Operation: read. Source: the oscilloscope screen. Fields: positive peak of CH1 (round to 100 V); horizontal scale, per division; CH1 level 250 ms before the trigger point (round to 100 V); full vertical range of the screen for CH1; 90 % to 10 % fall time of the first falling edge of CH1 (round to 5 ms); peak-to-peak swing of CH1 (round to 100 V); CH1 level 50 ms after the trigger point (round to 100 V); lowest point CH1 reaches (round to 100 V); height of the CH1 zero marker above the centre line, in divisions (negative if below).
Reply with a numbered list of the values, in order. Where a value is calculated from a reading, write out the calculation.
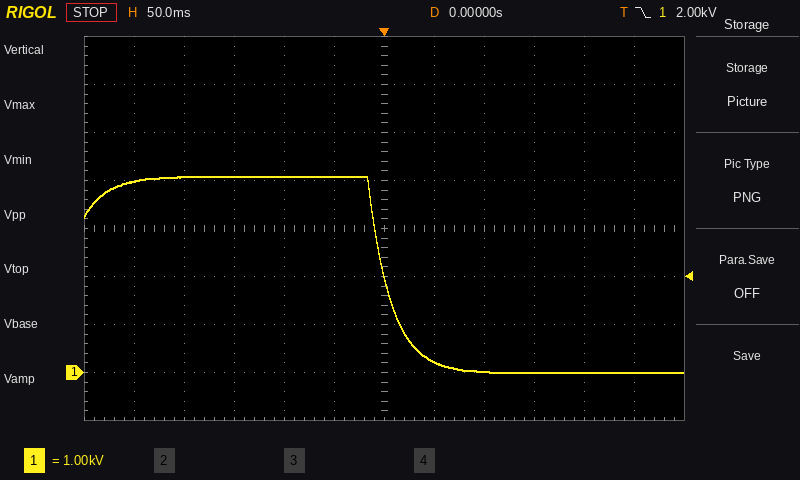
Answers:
1. 4.1 kV
2. 50 ms
3. 4.0 kV
4. 8 kV
5. 50 ms
6. 4.1 kV − (0.0 kV) = 4.1 kV
7. 200 V
8. 0.0 kV
9. -3.0 div
